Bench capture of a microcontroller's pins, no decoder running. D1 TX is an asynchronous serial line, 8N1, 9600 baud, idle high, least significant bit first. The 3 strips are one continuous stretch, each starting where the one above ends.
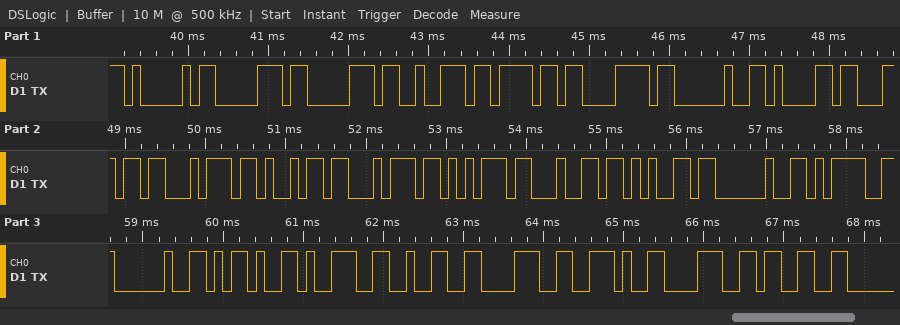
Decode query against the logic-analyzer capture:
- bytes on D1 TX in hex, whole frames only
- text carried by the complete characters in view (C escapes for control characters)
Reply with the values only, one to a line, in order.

0x41 0x70 0x70 0x72 0x6F 0x78 0x20 0x61 0x6C 0x74 0x69 0x74 0x75 0x64 0x65 0x20 0x3D 0x20 0x2D 0x39 0x32 0x38 0x2E 0x38 0x33
"Approx altitude = -928.83"
